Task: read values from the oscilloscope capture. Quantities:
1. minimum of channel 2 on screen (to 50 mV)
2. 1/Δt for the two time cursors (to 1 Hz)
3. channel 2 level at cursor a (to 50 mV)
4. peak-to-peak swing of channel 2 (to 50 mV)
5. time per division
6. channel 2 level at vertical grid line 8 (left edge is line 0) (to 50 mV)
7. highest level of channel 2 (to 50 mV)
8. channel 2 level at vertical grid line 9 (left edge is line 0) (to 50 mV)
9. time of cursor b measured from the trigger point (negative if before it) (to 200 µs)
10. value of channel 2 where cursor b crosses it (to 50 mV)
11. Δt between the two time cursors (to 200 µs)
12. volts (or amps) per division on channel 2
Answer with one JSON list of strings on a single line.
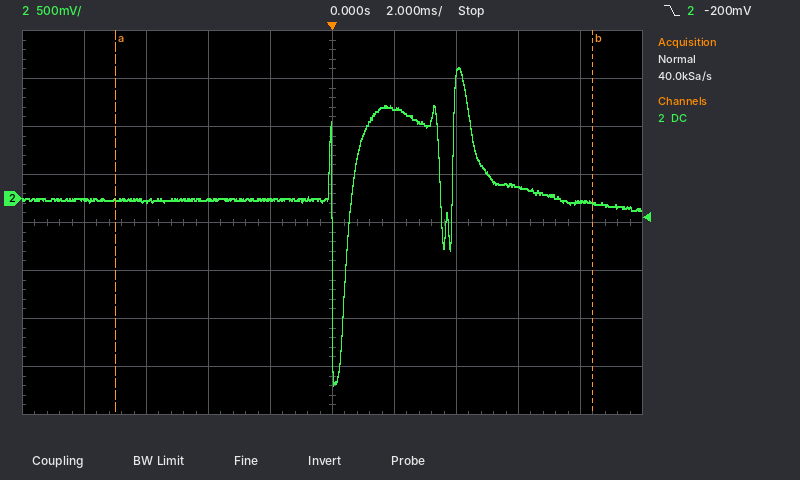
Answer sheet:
["-1.95 V", "65 Hz", "0 mV", "3.30 V", "2 ms", "100 mV", "1.35 V", "-50 mV", "+8.4 ms", "-50 mV", "15.4 ms", "500 mV"]
